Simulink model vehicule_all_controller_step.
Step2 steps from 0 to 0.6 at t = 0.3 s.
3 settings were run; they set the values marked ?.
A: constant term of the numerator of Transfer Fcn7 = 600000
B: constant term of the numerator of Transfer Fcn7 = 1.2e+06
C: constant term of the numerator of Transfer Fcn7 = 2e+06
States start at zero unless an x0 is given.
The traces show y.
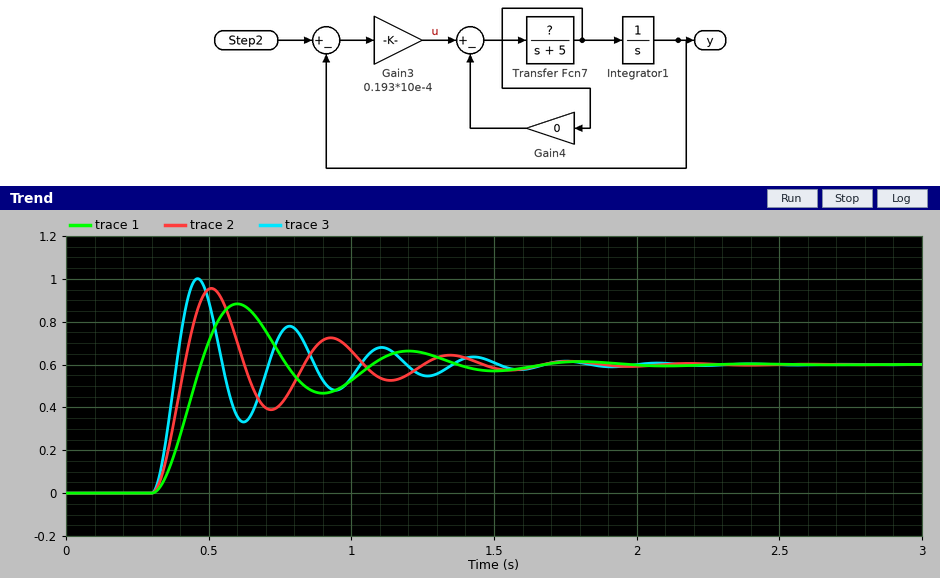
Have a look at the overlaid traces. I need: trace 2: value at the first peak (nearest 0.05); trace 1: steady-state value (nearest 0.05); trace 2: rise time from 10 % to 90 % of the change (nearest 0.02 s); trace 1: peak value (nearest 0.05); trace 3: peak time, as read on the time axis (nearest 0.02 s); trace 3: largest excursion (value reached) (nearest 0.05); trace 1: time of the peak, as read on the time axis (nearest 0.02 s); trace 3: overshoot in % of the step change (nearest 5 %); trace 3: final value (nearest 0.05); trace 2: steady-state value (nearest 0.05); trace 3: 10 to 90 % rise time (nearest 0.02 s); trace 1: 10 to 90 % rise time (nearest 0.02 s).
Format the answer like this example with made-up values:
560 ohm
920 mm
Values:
0.95
0.60
0.08 s
0.90
0.46 s
1.00
0.60 s
65 %
0.60
0.60
0.06 s
0.12 s
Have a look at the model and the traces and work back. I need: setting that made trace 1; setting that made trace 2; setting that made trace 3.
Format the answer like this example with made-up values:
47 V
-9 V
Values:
A
B
C
